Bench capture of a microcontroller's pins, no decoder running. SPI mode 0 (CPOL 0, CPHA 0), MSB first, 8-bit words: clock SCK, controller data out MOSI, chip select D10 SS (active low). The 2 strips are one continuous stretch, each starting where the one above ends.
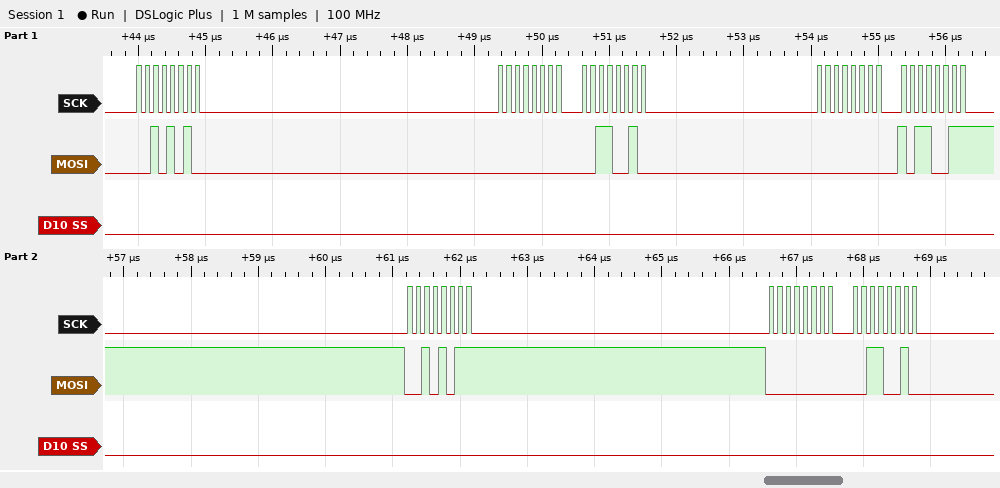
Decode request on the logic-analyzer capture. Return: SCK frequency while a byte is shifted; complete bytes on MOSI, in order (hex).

8 MHz
2A 00 32 00 B3 2B 00 32
